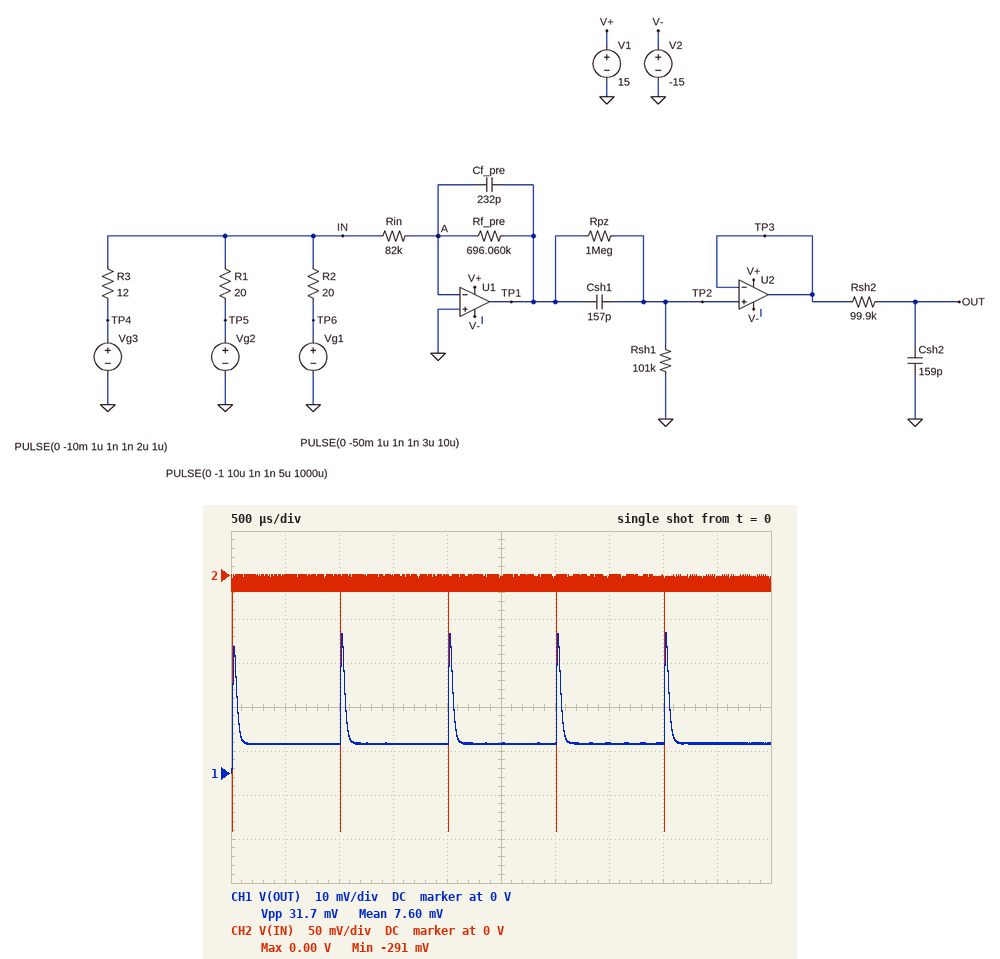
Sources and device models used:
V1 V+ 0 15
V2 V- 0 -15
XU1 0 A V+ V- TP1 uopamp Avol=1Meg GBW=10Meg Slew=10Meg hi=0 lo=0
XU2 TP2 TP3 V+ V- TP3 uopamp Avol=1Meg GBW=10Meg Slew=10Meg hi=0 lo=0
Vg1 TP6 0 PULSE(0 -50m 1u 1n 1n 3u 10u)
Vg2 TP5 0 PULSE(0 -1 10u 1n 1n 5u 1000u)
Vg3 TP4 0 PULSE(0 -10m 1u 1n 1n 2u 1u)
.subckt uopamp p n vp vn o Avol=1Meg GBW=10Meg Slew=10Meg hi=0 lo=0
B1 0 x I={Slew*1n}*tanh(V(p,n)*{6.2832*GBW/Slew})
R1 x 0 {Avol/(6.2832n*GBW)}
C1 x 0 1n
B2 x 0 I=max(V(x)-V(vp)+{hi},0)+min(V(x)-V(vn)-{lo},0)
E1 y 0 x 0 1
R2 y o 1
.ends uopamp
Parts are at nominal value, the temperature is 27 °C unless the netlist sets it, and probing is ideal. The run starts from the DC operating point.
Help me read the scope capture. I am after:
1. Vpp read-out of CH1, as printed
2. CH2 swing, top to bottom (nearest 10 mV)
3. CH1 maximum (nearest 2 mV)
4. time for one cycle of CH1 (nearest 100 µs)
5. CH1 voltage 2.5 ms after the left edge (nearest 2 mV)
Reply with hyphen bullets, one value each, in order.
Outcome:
- 31.7 mV
- 290 mV
- 32 mV
- 1.0 ms
- 6 mV
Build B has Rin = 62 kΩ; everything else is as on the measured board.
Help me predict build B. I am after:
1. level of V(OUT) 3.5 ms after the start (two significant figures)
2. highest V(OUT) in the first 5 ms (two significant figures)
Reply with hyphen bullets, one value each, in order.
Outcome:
- 8.9 mV
- 42 mV
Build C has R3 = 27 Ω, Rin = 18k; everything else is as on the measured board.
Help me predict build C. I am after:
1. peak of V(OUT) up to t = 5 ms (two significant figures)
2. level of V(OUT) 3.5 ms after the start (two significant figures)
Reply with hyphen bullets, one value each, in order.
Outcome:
- 180 mV
- 29 mV
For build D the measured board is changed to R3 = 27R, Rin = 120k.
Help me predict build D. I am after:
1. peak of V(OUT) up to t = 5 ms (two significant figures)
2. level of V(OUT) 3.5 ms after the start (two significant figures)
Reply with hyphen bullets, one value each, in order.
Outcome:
- 27 mV
- 4.4 mV
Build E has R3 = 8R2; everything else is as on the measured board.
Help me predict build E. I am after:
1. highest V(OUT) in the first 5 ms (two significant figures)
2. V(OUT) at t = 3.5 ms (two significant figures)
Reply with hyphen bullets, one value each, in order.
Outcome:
- 28 mV
- 6.9 mV
